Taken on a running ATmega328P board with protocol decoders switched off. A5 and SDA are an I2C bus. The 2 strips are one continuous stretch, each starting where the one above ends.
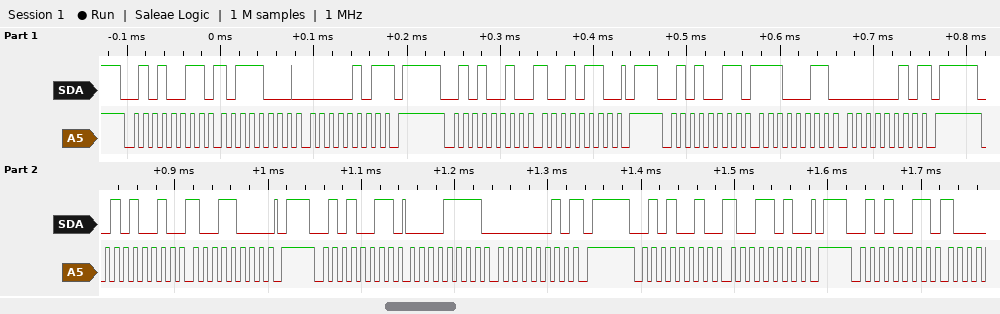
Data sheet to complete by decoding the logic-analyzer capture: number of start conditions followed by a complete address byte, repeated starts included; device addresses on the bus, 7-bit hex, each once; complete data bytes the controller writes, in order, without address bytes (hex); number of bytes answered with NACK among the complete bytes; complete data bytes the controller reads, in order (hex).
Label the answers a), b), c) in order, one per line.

a) 7
b) 0x29
c) 96 98 9A
d) 3
e) B8 05 E3 02 0F 02
